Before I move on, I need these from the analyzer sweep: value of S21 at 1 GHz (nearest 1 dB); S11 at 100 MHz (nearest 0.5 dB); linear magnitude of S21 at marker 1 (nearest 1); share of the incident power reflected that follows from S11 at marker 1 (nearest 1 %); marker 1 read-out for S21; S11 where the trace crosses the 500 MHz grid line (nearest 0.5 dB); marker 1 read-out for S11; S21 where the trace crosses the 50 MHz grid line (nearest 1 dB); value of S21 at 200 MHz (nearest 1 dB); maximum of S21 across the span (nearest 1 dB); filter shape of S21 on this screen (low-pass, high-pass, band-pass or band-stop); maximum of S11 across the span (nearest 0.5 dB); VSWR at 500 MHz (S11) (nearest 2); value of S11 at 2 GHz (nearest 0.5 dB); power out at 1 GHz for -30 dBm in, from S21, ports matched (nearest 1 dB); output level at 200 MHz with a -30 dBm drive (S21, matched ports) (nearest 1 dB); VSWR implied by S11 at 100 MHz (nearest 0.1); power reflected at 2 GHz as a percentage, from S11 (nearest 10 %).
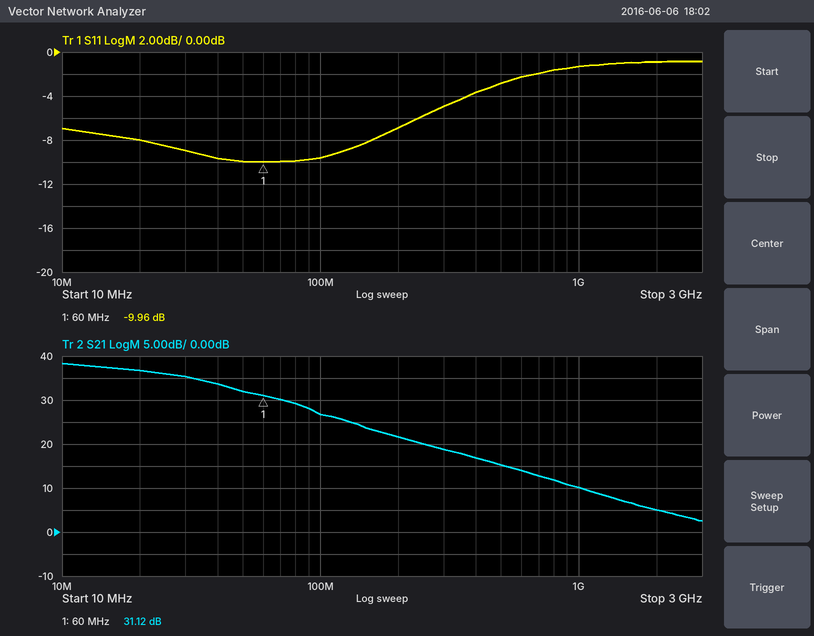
10 dB
-9.5 dB
36
10 %
31.12 dB
-3.0 dB
-9.96 dB
32 dB
22 dB
38 dB
low-pass
-1.0 dB
6
-1.0 dB
-20 dBm
-8 dBm
2.0
80 %
